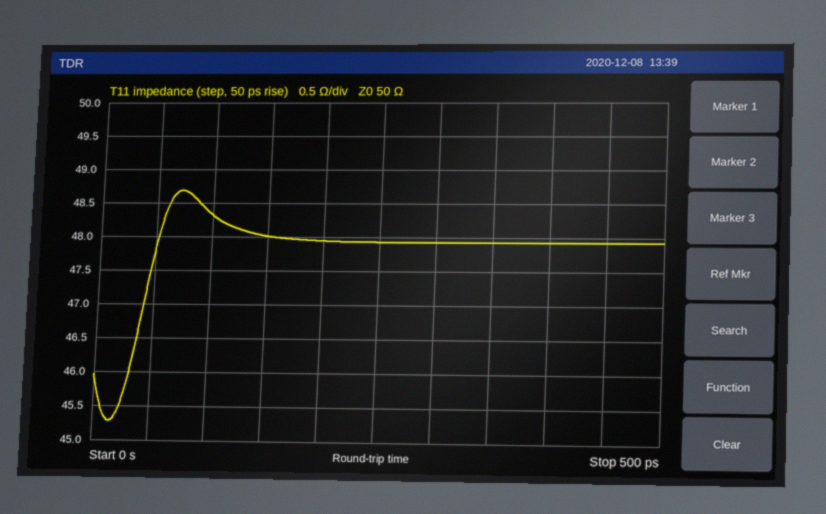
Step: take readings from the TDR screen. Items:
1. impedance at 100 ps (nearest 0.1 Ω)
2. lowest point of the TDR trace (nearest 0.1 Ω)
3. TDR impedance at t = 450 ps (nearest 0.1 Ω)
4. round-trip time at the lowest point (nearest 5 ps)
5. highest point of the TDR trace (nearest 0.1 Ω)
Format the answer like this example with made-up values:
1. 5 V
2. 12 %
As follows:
1. 48.3 Ω
2. 45.3 Ω
3. 47.9 Ω
4. 15 ps
5. 48.7 Ω
